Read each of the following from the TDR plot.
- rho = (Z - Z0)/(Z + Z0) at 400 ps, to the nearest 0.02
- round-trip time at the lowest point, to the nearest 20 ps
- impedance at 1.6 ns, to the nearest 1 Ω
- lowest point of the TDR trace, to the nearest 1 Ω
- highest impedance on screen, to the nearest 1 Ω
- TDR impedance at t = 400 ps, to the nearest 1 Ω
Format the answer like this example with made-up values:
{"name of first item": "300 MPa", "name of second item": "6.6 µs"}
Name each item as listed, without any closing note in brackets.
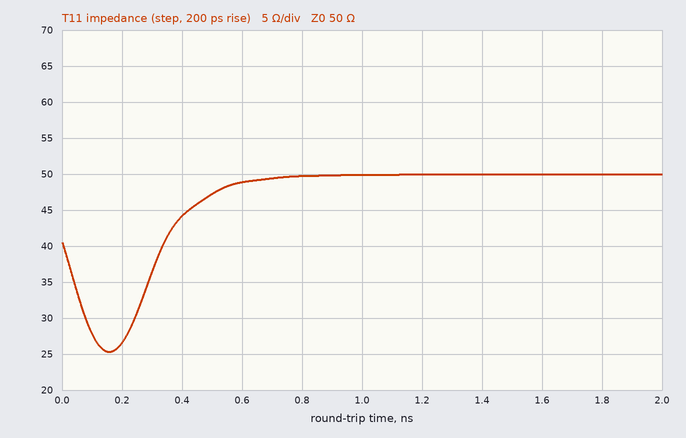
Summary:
{"rho = (Z - Z0)/(Z + Z0) at 400 ps, to the nearest 0.02": "-0.06", "round-trip time at the lowest point, to the nearest 20 ps": "160 ps", "impedance at 1.6 ns, to the nearest 1 Ω": "50 Ω", "lowest point of the TDR trace, to the nearest 1 Ω": "25 Ω", "highest impedance on screen, to the nearest 1 Ω": "50 Ω", "TDR impedance at t = 400 ps, to the nearest 1 Ω": "44 Ω"}
